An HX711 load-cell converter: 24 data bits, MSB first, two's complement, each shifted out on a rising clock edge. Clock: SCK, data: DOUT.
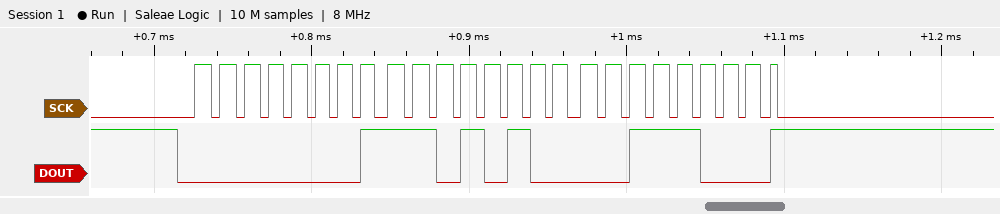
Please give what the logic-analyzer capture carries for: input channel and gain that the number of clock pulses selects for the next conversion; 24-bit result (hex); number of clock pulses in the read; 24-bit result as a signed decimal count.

channel A, gain 128
0x01D438
25
119864
